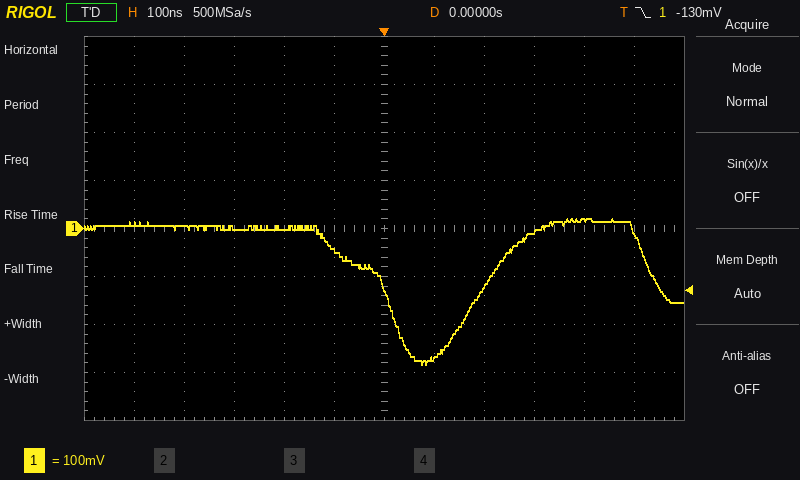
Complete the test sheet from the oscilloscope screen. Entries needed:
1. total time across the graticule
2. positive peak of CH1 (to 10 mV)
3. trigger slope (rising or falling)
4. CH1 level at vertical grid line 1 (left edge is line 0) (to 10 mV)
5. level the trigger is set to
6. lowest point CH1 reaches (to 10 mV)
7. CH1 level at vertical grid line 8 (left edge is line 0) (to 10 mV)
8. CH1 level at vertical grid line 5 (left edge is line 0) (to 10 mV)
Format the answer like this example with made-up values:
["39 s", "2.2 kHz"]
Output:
["1.2 µs", "20 mV", "falling", "10 mV", "-130 mV", "-280 mV", "-120 mV", "-50 mV"]
